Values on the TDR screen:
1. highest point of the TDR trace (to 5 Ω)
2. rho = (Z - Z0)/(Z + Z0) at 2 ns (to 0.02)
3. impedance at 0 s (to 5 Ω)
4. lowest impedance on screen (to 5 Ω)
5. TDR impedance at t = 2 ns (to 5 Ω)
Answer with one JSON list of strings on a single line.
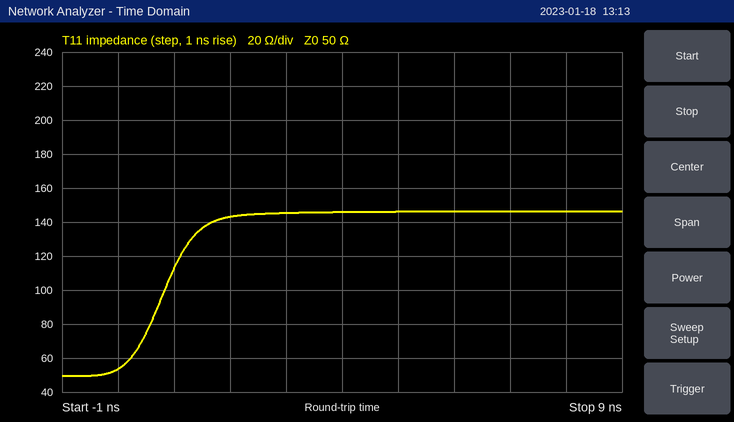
["145 Ω", "+0.48", "55 Ω", "50 Ω", "145 Ω"]
